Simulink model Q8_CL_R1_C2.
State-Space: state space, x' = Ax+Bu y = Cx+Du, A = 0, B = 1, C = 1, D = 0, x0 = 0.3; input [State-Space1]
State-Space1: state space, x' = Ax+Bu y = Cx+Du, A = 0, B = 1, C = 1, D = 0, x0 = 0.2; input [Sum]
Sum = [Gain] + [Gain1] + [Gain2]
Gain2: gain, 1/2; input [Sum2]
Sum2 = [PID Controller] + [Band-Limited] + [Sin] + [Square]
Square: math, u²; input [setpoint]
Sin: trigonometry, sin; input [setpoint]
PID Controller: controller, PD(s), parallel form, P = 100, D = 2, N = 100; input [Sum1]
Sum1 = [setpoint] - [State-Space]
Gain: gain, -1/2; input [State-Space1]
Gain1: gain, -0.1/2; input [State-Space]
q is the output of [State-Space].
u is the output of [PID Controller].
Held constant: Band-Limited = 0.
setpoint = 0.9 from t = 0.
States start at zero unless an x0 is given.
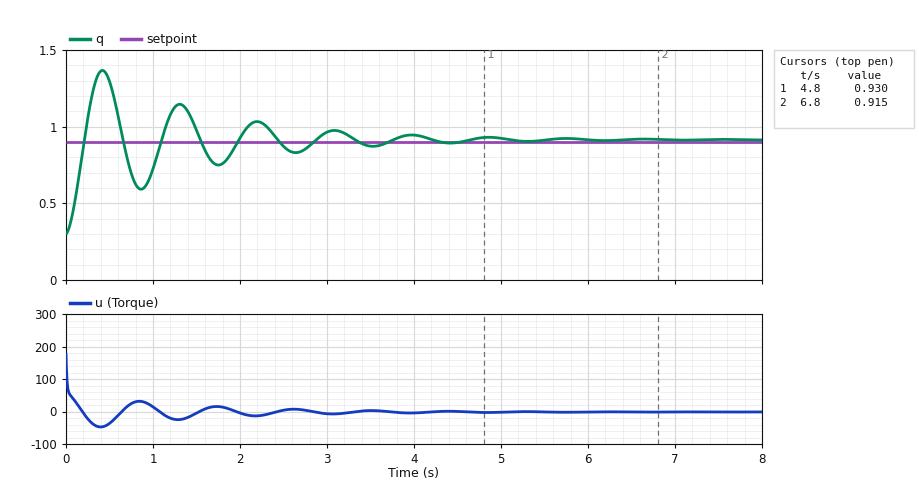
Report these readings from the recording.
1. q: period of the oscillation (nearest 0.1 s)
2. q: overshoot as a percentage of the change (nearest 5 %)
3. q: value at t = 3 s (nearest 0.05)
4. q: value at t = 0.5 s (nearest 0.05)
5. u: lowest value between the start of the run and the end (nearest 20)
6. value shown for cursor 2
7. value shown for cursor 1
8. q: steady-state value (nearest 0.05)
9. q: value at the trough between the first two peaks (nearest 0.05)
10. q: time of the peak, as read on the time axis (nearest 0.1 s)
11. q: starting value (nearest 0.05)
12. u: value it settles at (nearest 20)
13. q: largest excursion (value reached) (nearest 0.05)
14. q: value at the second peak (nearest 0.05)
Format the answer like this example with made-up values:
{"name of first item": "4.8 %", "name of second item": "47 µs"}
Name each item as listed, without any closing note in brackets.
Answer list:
{"q: period of the oscillation": "0.9 s", "q: overshoot as a percentage of the change": "75 %", "q: value at t = 3 s": "0.95", "q: value at t = 0.5 s": "1.30", "u: lowest value between the start of the run and the end": "-40", "value shown for cursor 2": "0.915", "value shown for cursor 1": "0.930", "q: steady-state value": "0.90", "q: value at the trough between the first two peaks": "0.60", "q: time of the peak, as read on the time axis": "0.4 s", "q: starting value": "0.30", "u: value it settles at": "0", "q: largest excursion (value reached)": "1.35", "q: value at the second peak": "1.15"}
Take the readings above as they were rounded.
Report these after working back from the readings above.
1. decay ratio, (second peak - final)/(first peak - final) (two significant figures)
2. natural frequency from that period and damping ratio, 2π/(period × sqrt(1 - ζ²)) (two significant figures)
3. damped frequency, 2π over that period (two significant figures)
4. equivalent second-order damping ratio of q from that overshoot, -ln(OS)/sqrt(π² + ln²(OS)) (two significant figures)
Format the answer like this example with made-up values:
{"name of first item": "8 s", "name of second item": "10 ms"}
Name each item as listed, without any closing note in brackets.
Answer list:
{"decay ratio, (second peak - final)/(first peak - final)": "0.56", "natural frequency from that period and damping ratio, 2π/(period × sqrt(1 - ζ²))": "7.0 rad/s", "damped frequency, 2π over that period": "7.0 rad/s", "equivalent second-order damping ratio of q from that overshoot, -ln(OS)/sqrt(π² + ln²(OS))": "0.091"}
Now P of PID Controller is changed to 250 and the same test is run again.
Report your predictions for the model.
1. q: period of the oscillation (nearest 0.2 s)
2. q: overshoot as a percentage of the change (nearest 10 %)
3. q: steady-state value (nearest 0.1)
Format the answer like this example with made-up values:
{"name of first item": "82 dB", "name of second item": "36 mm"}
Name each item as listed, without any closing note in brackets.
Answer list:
{"q: period of the oscillation": "0.6 s", "q: overshoot as a percentage of the change": "80 %", "q: steady-state value": "0.9"}
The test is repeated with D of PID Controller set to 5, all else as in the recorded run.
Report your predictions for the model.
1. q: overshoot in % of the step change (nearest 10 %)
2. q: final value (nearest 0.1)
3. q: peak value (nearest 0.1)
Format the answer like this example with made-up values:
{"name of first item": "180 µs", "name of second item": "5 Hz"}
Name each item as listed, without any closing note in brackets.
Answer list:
{"q: overshoot in % of the step change": "60 %", "q: final value": "0.9", "q: peak value": "1.3"}
